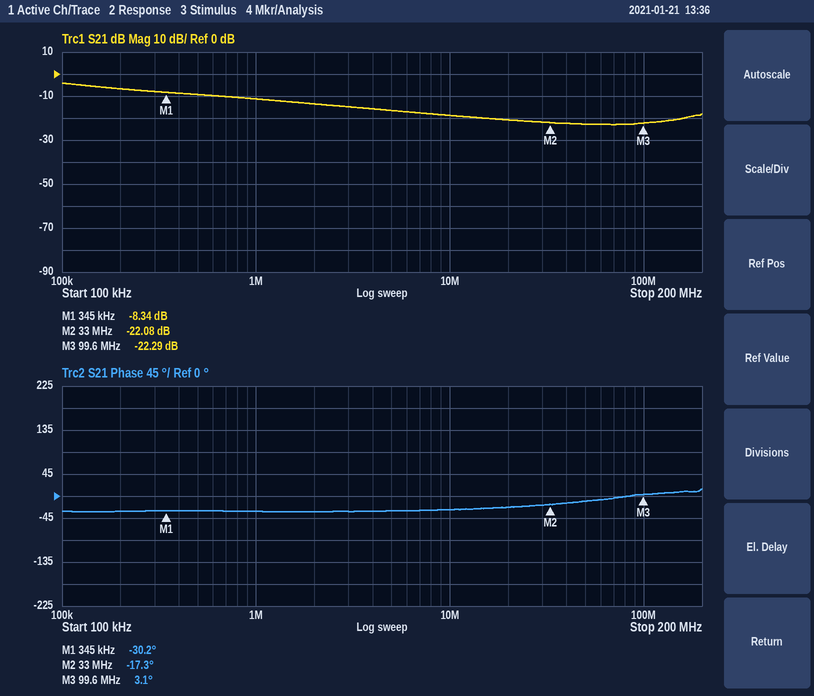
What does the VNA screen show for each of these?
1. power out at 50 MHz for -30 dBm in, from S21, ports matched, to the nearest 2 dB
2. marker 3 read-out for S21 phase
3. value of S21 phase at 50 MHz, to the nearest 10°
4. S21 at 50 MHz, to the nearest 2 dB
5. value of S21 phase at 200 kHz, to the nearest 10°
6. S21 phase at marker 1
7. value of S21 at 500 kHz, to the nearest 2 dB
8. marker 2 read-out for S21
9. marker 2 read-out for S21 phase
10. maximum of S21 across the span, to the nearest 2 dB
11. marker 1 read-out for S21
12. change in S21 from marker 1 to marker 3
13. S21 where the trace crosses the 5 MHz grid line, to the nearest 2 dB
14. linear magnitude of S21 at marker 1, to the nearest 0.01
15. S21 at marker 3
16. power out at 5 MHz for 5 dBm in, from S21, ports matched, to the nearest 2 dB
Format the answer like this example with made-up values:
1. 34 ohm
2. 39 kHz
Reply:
1. -52 dBm
2. 3.1°
3. -10°
4. -22 dB
5. -30°
6. -30.2°
7. -10 dB
8. -22.08 dB
9. -17.3°
10. -4 dB
11. -8.34 dB
12. -13.95 dB
13. -16 dB
14. 0.38
15. -22.29 dB
16. -12 dBm
